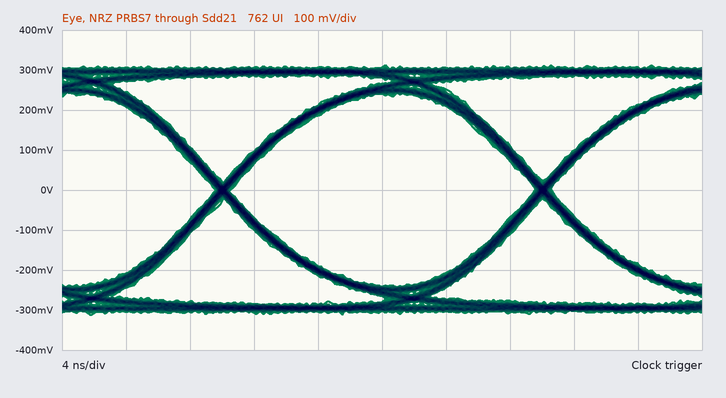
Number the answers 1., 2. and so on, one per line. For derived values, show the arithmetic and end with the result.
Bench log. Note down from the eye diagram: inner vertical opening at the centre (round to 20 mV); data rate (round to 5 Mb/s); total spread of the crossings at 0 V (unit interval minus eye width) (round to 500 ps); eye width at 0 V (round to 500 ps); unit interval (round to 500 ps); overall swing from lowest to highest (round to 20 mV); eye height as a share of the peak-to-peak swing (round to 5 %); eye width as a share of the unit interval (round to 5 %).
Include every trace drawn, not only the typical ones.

1. 480 mV
2. 50 Mb/s
3. 1.0 ns
4. 19.0 ns
5. 20.0 ns
6. 620 mV
7. 480 mV / 620 mV ≈ 77.4 %, so 75 % to the nearest 5 %
8. 19.0 ns / 20.0 ns ≈ 95 %
